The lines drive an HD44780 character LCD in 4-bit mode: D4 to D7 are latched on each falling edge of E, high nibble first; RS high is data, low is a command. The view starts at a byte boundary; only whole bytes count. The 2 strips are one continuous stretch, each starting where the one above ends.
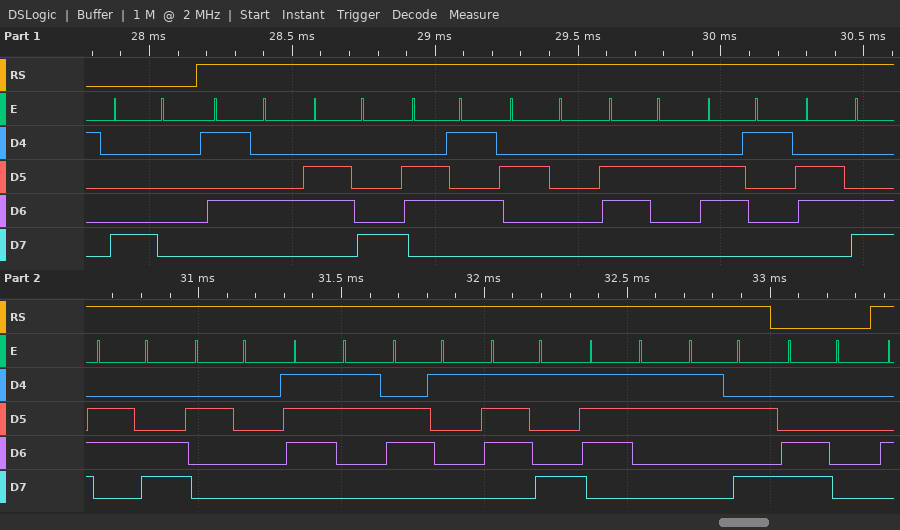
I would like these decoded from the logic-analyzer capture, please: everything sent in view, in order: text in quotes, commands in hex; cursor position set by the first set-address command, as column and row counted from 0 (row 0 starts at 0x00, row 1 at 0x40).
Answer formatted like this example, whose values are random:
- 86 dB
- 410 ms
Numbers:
- 0x80 "The ball says:" 0xC0
- column 0, row 0
